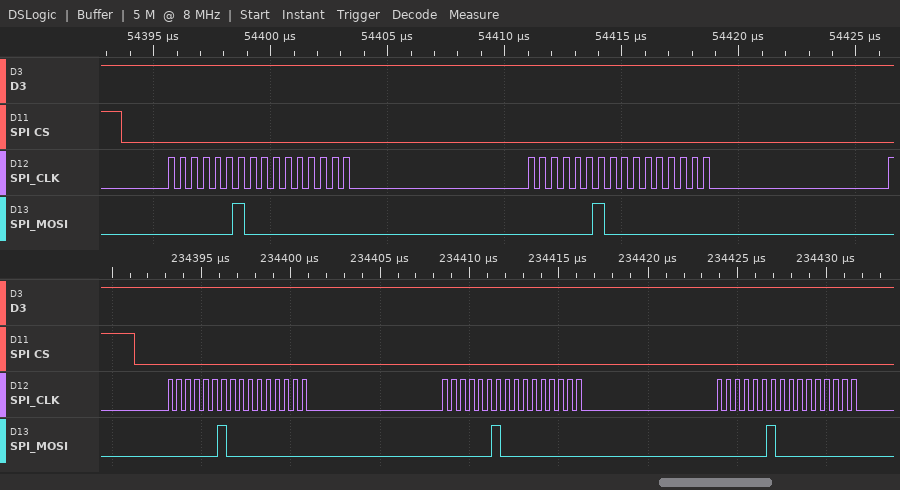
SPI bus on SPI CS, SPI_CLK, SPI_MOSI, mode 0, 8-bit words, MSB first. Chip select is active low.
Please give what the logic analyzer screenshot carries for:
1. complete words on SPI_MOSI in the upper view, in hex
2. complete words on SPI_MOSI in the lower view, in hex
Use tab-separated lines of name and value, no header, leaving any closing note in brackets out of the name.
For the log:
complete words on SPI_MOSI in the upper view, in hex	02, 00, 02, 00
complete words on SPI_MOSI in the lower view, in hex	02, 00, 02, 00, 02, 00
